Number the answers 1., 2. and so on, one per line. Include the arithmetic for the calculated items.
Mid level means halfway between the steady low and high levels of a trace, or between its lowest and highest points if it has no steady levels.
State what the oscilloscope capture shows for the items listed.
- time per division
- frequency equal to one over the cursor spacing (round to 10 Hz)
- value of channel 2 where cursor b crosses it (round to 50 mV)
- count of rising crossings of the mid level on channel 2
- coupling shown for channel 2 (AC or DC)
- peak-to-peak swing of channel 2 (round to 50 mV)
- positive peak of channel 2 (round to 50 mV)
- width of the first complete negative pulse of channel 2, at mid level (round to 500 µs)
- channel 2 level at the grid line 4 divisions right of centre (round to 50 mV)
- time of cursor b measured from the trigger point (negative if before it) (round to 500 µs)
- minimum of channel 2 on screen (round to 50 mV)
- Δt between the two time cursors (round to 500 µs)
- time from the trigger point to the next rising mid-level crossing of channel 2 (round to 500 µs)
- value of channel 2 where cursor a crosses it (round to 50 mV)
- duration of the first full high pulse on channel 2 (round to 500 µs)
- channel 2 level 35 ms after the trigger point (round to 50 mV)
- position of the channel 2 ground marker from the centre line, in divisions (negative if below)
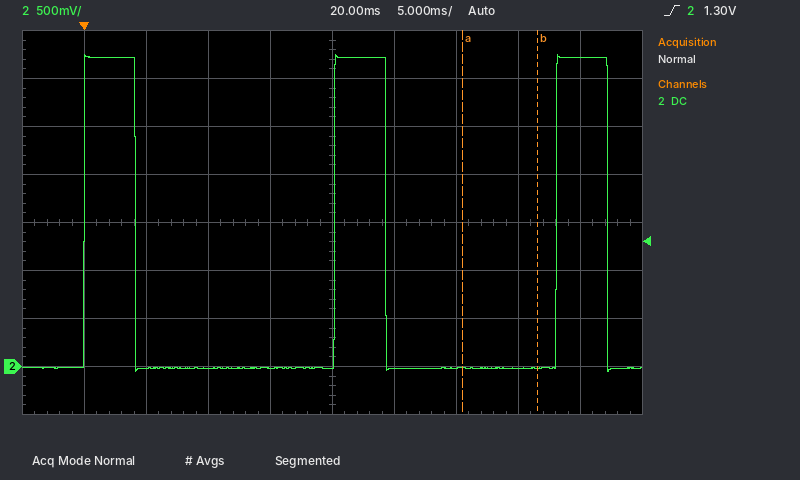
1. 5 ms
2. 1 / 6.0 ms ≈ 170 Hz
3. 0 mV
4. 3
5. DC
6. 3.25 V − (-50 mV) = 3.30 V
7. 3.25 V
8. 16.0 ms
9. 3.20 V
10. +36.5 ms
11. -50 mV
12. 6.0 ms
13. 20.0 ms
14. 0 mV
15. 4.0 ms
16. 0 mV
17. -3.0 div
